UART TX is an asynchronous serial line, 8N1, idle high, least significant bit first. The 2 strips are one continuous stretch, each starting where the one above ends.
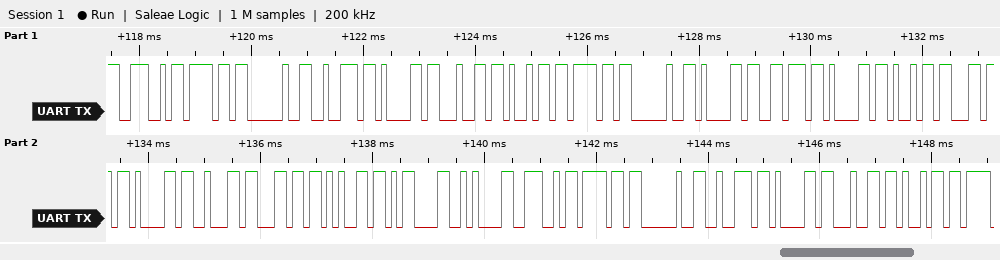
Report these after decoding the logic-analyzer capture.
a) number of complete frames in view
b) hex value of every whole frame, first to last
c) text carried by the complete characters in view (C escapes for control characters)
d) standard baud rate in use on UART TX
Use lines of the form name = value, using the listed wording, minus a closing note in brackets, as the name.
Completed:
number of complete frames in view = 27
hex value of every whole frame, first to last = 4E 6F 20 72 61 64 69 6F 20 61 76 61 69 6C 61 62 6C 65 0D 0A 4E 6F 20 72 61 64 69
text carried by the complete characters in view = "No radio available\r\nNo radi"
standard baud rate in use on UART TX = 9600 baud
